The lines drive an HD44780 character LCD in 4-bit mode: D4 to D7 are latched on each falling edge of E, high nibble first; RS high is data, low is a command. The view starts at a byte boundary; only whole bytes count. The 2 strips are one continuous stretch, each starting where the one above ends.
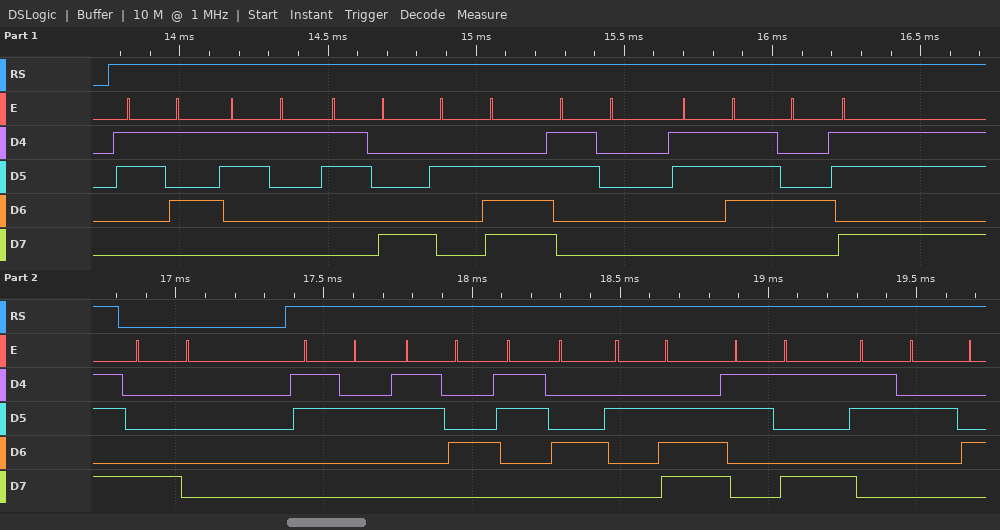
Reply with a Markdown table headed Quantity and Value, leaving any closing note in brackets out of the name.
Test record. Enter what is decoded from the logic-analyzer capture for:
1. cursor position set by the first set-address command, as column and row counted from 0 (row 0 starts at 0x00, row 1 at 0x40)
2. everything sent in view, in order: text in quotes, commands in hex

| Quantity | Value |
|---|---|
| cursor position set by the first set-address command, as column and row counted from 0 | column 0, row 0 |
| everything sent in view, in order: text in quotes, commands in hex | "518.07K" 0x80 "244.92" |
